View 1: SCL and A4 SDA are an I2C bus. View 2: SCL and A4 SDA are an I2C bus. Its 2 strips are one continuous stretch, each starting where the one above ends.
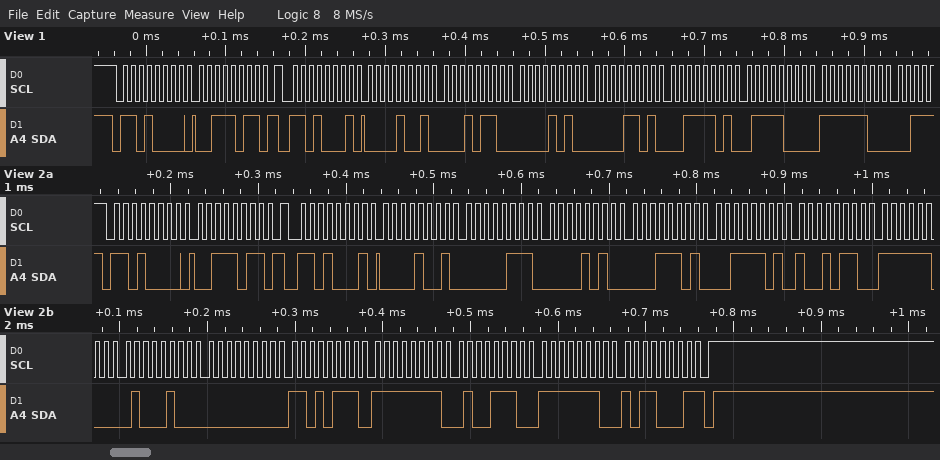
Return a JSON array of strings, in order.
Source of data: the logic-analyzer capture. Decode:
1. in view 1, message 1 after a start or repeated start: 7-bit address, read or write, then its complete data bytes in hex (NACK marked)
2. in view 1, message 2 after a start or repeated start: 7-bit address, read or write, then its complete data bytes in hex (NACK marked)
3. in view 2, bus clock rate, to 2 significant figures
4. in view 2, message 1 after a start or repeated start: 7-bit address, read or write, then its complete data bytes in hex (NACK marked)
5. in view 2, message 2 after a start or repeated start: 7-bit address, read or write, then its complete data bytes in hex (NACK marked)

["0x68 write: 3B", "0x68 read: 09 16 0A 0D 3D 78 FC", "100 kHz", "0x68 write: 3B", "0x68 read: 09 07 0A 1D 3D 96 FC 44 00 D7 FF 4E FE B1 NACK"]
